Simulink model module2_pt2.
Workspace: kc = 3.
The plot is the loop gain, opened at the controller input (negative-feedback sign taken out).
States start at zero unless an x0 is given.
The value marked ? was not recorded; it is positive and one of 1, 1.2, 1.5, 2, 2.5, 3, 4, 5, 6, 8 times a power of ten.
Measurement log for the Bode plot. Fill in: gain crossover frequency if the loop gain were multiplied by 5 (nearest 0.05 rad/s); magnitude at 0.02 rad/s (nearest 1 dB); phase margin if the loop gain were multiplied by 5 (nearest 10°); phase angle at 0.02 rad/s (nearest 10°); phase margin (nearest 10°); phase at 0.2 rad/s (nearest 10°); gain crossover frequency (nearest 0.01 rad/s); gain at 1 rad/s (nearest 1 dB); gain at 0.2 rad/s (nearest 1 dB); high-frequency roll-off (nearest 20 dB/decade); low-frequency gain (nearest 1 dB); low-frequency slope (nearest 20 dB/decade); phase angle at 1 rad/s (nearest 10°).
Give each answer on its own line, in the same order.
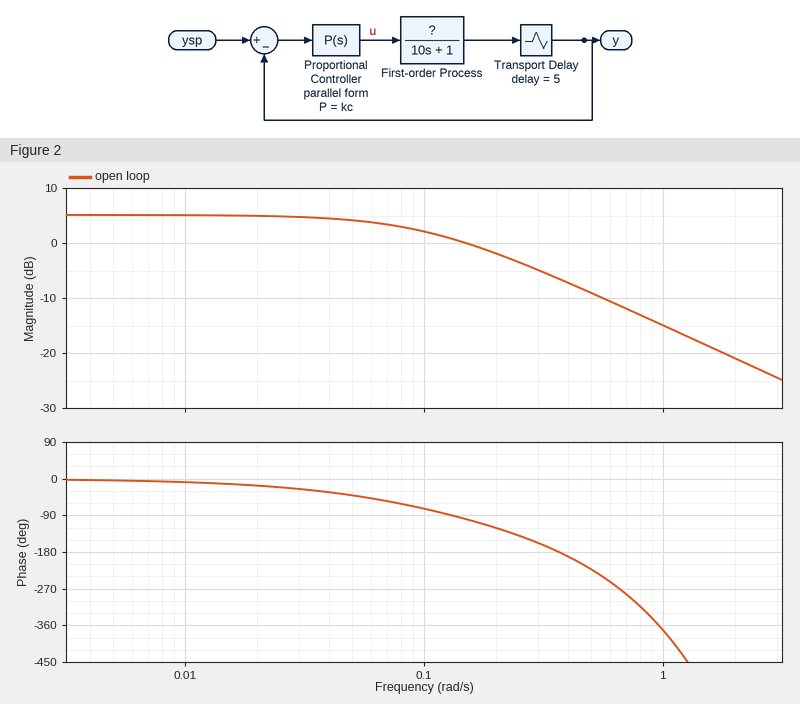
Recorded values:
0.90 rad/s
5 dB
-160°
-20°
80°
-120°
0.15 rad/s
-15 dB
-2 dB
-20 dB/decade
5 dB
0 dB/decade
-370°
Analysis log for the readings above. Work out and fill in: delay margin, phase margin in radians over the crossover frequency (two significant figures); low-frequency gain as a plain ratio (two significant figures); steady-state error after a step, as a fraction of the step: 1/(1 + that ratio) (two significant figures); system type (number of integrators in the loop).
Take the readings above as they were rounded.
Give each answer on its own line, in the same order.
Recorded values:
9.3 s
1.8
0.36
0
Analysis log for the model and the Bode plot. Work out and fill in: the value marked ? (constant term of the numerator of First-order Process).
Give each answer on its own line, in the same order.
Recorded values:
0.6
